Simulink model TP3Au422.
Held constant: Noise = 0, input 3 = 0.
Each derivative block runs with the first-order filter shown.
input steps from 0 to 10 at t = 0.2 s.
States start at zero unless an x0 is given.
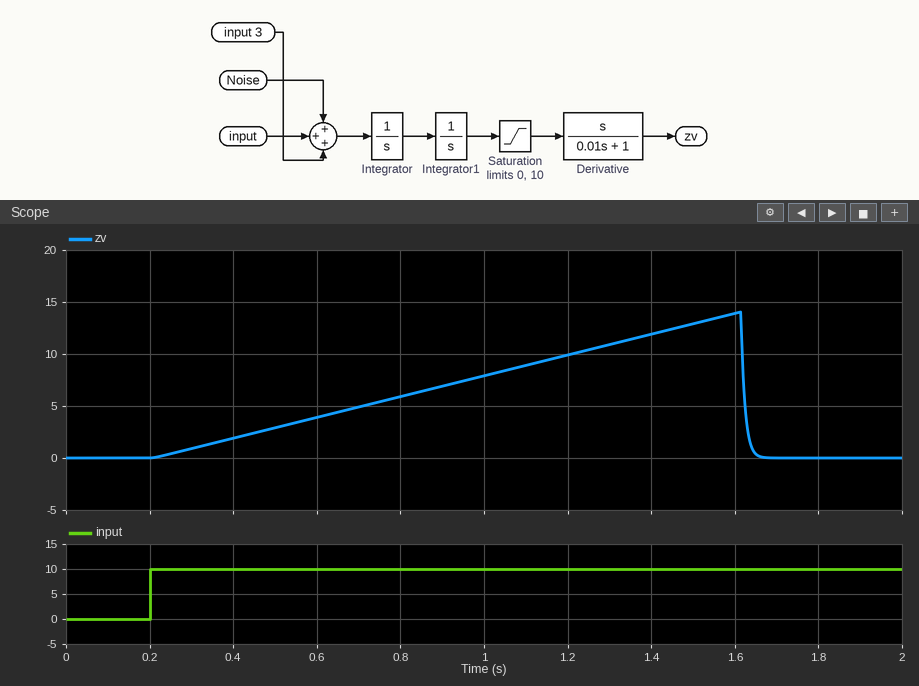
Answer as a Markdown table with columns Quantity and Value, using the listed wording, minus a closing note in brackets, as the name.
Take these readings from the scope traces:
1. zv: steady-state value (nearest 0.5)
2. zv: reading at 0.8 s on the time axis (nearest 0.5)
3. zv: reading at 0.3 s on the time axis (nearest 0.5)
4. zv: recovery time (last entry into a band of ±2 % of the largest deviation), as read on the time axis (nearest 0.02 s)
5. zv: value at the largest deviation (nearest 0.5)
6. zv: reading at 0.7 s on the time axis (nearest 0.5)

| Quantity | Value |
|---|---|
| zv: steady-state value | 0.0 |
| zv: reading at 0.8 s on the time axis | 6.0 |
| zv: reading at 0.3 s on the time axis | 1.0 |
| zv: recovery time (last entry into a band of ±2 % of the largest deviation), as read on the time axis | 1.66 s |
| zv: value at the largest deviation | 14.0 |
| zv: reading at 0.7 s on the time axis | 5.0 |
